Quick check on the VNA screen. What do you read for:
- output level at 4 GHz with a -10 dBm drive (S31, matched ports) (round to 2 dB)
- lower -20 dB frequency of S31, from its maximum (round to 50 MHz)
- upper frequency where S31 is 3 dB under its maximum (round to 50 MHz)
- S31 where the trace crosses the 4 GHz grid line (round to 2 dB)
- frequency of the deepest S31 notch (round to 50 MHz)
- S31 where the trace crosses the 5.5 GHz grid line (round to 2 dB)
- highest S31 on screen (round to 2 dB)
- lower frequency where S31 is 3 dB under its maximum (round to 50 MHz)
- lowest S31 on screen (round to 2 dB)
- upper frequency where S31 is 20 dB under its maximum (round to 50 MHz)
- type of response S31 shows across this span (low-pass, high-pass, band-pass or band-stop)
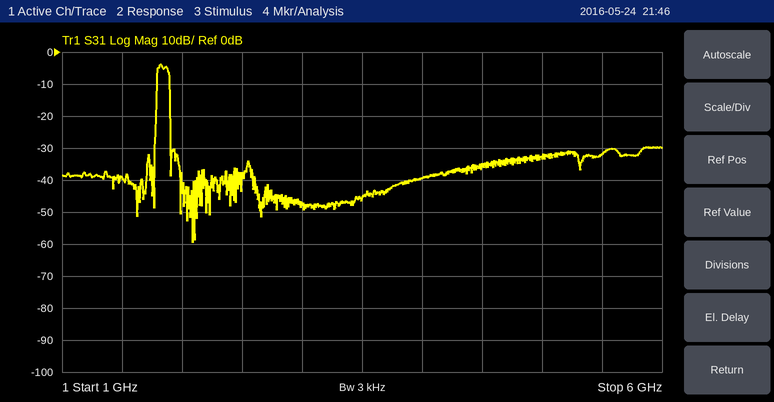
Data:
-50 dBm
1.80 GHz
1.90 GHz
-40 dB
2.10 GHz
-32 dB
-4 dB
1.80 GHz
-60 dB
1.90 GHz
band-pass
